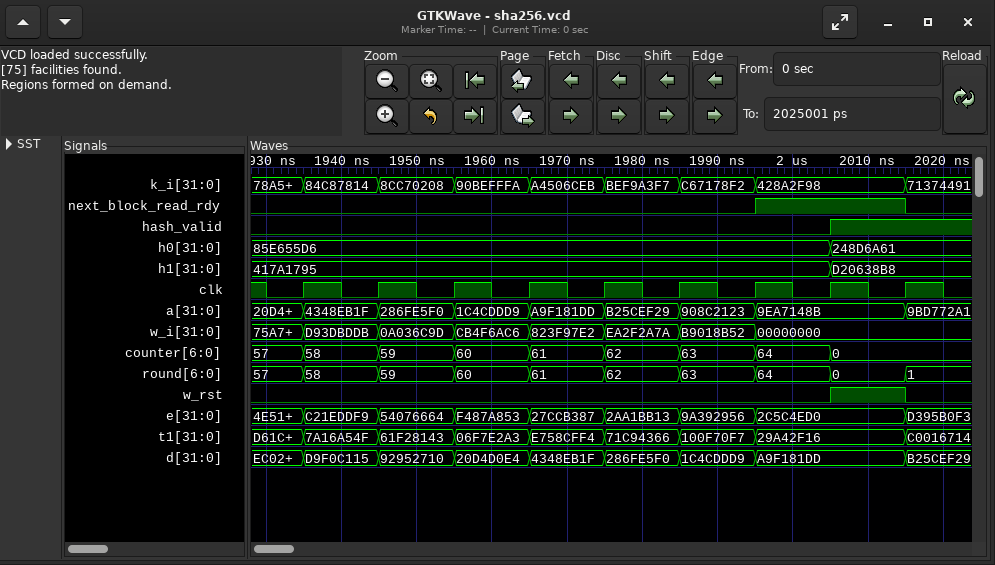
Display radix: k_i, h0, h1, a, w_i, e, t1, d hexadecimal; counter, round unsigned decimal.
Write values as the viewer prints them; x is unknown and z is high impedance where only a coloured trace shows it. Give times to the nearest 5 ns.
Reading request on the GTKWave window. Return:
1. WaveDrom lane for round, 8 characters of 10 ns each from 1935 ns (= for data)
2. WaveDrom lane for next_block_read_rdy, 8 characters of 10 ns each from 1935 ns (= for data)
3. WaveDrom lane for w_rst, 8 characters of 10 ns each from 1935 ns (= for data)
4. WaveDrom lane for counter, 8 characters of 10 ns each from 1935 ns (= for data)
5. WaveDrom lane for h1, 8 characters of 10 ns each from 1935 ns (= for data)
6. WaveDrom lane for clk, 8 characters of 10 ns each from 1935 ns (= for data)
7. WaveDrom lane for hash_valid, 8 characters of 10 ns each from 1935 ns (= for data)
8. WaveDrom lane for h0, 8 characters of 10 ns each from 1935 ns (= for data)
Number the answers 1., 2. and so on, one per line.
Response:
1. {name: 'round', wave: '========', data: '58 59 60 61 62 63 64 0'}
2. {name: 'next_block_read_rdy', wave: '0.....1.'}
3. {name: 'w_rst', wave: '0......1'}
4. {name: 'counter', wave: '========', data: '58 59 60 61 62 63 64 0'}
5. {name: 'h1', wave: '=......=', data: '417A1795 D20638B8'}
6. {name: 'clk', wave: 'p.......'}
7. {name: 'hash_valid', wave: '0......1'}
8. {name: 'h0', wave: '=......=', data: '85E655D6 248D6A61'}
